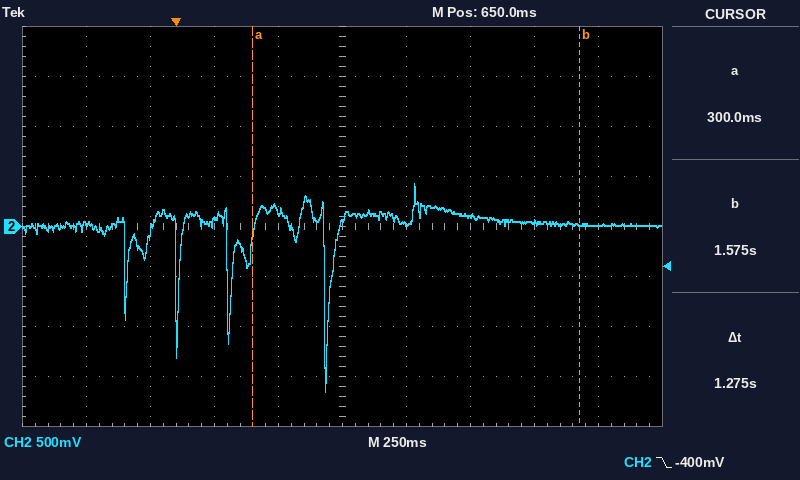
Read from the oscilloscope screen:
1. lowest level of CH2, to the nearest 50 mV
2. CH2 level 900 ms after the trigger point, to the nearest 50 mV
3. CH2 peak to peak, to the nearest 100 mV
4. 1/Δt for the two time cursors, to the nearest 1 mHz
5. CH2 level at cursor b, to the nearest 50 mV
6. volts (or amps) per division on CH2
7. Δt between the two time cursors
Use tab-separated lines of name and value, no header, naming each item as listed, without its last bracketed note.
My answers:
lowest level of CH2, to the nearest 50 mV	-1.65 V
CH2 level 900 ms after the trigger point, to the nearest 50 mV	50 mV
CH2 peak to peak, to the nearest 100 mV	2.10 V
1/Δt for the two time cursors, to the nearest 1 mHz	784 mHz
CH2 level at cursor b, to the nearest 50 mV	0 mV
volts (or amps) per division on CH2	500 mV
Δt between the two time cursors	1.275 s
